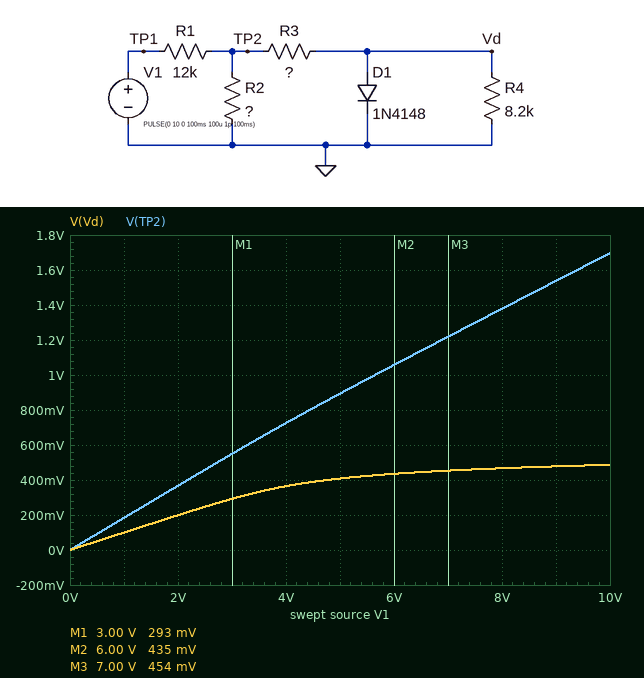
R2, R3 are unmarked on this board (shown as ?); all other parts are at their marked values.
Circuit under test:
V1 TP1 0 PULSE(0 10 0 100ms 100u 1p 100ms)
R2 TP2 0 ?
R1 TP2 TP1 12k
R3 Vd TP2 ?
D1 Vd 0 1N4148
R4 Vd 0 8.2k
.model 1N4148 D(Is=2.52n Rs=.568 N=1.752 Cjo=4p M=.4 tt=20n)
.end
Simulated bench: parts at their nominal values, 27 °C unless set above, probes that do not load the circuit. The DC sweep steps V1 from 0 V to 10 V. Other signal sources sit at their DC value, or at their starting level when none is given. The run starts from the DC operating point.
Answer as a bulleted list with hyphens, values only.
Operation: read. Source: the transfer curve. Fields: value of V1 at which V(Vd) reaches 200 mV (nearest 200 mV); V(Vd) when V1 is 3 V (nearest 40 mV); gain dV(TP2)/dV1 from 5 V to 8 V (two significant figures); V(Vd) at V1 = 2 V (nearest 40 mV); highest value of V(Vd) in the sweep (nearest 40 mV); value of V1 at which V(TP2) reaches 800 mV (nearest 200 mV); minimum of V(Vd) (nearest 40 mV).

- 2.0 V
- 280 mV
- 0.16 V/V
- 200 mV
- 480 mV
- 4.4 V
- 0 V
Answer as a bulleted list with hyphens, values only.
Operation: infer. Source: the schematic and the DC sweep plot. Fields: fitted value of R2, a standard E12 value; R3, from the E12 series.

- 3.3 kΩ
- 6.8 kΩ
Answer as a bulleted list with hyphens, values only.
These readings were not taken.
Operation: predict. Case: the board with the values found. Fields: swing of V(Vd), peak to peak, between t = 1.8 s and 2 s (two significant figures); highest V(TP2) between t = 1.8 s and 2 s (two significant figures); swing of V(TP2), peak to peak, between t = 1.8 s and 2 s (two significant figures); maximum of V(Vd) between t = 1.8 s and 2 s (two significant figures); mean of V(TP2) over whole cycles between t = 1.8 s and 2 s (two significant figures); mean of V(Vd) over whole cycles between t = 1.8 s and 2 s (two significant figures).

- 490 mV
- 1.7 V
- 1.7 V
- 490 mV
- 880 mV
- 350 mV
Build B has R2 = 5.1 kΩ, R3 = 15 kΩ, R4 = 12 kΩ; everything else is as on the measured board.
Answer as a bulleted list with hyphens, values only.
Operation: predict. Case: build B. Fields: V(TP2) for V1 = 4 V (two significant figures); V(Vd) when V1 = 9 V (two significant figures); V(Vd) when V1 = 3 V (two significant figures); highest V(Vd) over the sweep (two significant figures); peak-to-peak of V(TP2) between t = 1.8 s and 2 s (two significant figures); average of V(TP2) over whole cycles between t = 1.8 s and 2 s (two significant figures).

- 1.0 V
- 470 mV
- 330 mV
- 480 mV
- 2.5 V
- 1.3 V
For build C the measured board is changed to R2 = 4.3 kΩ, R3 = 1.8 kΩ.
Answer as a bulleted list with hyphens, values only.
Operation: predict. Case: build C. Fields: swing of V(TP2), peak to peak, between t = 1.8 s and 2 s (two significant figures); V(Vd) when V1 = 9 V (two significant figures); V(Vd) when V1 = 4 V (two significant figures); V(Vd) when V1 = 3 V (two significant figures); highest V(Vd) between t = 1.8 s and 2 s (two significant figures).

- 1.3 V
- 530 mV
- 460 mV
- 420 mV
- 540 mV
